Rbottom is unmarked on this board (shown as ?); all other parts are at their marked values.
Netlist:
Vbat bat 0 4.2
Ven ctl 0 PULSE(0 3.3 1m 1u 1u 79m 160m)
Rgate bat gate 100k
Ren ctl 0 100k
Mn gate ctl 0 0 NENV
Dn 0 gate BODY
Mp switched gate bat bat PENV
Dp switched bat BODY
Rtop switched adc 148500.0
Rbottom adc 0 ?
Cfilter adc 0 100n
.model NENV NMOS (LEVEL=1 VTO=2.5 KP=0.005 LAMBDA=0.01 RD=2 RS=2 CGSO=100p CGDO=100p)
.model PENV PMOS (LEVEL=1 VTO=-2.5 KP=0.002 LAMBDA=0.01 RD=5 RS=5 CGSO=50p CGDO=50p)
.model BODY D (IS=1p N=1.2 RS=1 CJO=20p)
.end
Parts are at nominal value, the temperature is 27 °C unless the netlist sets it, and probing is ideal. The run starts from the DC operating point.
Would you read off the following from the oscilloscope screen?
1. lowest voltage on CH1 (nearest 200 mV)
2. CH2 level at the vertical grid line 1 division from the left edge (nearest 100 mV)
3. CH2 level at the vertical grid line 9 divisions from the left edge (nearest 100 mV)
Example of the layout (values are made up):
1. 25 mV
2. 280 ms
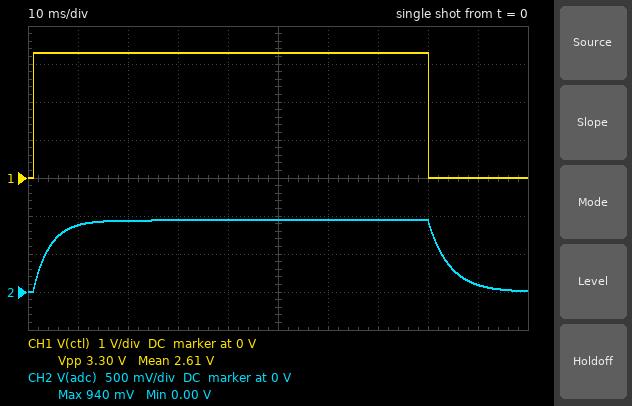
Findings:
1. 0 V
2. 900 mV
3. 100 mV
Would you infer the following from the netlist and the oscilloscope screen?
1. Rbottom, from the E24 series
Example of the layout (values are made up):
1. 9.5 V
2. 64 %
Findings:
1. 43 kΩ
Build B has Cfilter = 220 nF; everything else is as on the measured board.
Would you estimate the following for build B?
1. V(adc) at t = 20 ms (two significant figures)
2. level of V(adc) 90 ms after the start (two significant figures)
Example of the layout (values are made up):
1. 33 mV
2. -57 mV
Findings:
1. 870 mV
2. 330 mV
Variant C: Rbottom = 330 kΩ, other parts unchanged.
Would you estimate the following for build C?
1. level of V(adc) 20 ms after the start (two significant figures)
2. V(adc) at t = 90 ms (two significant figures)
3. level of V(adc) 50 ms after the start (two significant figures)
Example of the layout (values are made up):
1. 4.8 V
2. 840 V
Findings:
1. 2.4 V
2. 2.1 V
3. 2.9 V
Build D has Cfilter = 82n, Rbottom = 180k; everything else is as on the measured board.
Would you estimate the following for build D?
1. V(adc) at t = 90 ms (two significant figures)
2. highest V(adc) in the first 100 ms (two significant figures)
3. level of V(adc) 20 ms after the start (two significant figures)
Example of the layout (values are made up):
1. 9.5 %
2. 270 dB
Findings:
1. 1.2 V
2. 2.3 V
3. 2.2 V
